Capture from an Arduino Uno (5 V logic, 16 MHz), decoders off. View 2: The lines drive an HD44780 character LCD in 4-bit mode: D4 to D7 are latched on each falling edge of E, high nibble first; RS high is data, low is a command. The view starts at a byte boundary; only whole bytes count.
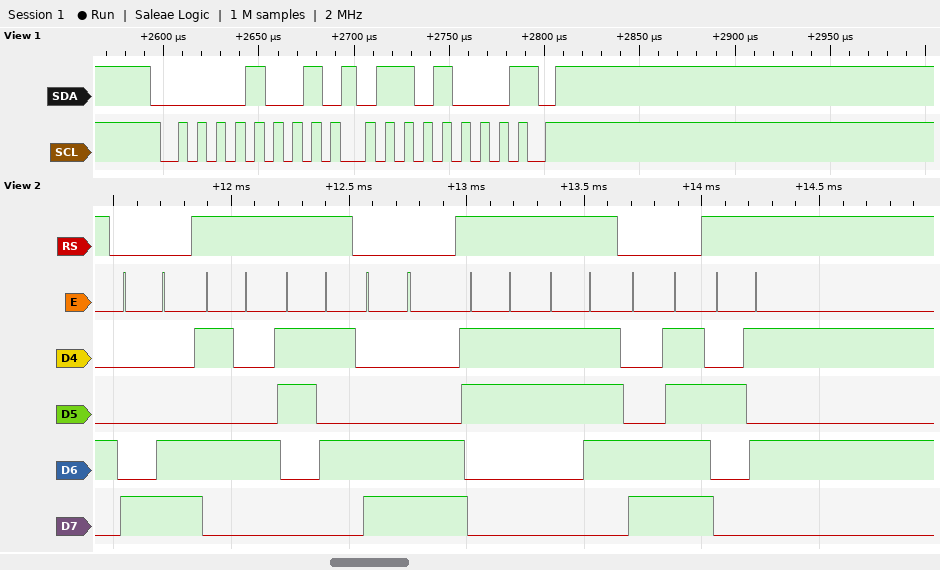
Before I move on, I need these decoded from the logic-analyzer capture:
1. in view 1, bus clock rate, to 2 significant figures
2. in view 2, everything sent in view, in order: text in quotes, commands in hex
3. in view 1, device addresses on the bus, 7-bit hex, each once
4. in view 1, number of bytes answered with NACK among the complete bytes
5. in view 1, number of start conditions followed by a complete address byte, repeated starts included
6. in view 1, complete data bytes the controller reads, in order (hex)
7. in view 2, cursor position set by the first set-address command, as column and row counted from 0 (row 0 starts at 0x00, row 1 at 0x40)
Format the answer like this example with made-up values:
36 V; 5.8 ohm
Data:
100 kHz; 0x8C "T5" 0xCC "37" 0xCF "%"; 0x04; 1; 1; 68; column 12, row 0
